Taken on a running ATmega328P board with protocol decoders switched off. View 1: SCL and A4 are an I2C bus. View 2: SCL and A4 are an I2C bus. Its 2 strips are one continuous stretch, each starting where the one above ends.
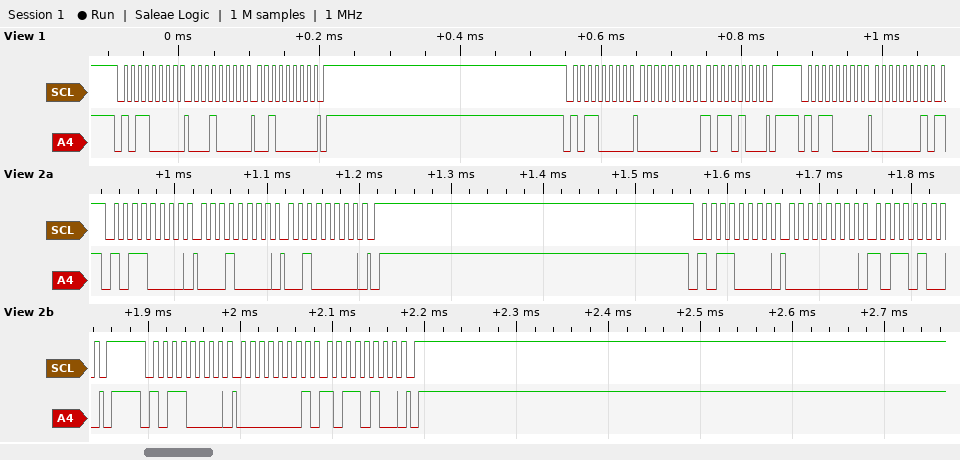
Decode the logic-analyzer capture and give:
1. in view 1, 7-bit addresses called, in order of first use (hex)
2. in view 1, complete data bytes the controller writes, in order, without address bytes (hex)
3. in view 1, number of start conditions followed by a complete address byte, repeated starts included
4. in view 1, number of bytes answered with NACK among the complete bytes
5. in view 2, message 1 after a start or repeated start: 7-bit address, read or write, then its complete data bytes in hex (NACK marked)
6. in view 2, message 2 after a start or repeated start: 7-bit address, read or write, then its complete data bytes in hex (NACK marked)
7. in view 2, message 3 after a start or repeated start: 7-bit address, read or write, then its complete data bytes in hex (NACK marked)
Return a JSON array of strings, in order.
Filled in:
["0x58", "10 20 00 B4 01", "3", "0", "0x58 write: 10 20", "0x58 write: 00 B4", "0x58 write: 01 B4"]
